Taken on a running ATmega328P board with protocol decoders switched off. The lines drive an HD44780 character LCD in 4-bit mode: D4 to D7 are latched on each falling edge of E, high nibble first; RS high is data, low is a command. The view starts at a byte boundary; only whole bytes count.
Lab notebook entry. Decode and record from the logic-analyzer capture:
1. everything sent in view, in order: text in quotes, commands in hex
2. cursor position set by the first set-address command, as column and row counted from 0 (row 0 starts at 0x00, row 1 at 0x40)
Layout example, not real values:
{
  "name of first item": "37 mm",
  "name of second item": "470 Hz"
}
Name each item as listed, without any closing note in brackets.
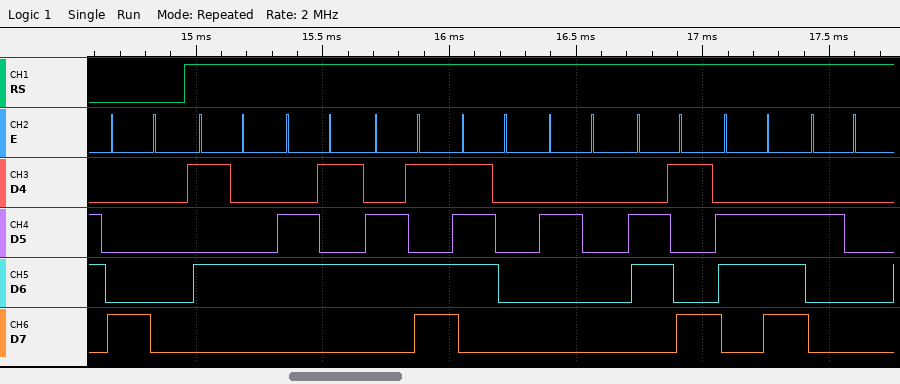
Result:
{
  "everything sent in view, in order: text in quotes, commands in hex": "0x80 \"Temp in \"",
  "cursor position set by the first set-address command, as column and row counted from 0": "column 0, row 0"
}
